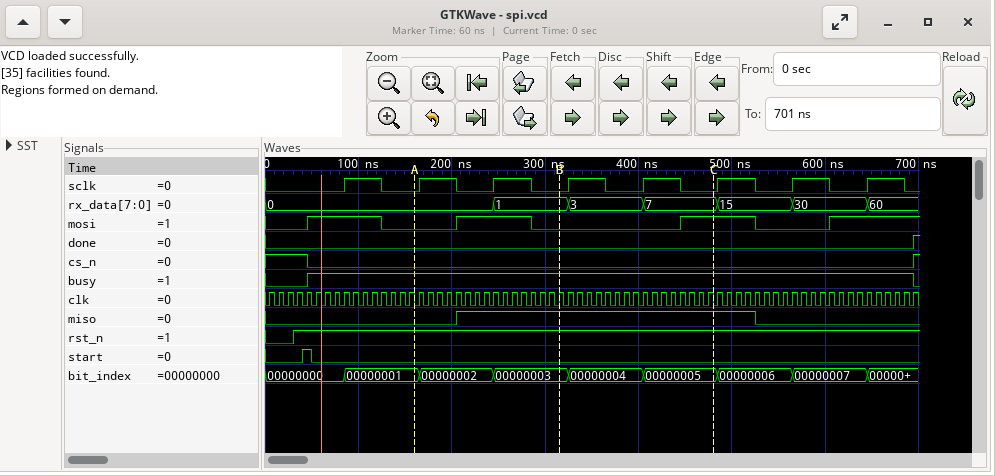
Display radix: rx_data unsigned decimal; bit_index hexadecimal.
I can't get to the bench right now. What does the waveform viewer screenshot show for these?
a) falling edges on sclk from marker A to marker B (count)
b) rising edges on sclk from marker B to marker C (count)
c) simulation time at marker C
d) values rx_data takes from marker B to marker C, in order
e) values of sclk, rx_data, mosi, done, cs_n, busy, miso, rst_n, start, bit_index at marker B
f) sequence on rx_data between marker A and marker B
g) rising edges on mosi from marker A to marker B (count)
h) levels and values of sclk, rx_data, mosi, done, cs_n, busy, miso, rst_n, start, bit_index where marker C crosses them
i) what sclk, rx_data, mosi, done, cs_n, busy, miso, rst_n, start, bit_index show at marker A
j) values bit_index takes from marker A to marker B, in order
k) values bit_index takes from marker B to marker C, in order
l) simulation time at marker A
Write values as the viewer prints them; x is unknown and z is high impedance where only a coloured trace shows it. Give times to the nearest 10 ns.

2
2
480 ns
1, 3, 7
sclk=0, rx_data=1, mosi=0, done=0, cs_n=0, busy=1, miso=1, rst_n=1, start=0, bit_index=00000003
0, 1
1
sclk=0, rx_data=7, mosi=1, done=0, cs_n=0, busy=1, miso=1, rst_n=1, start=0, bit_index=00000005
sclk=0, rx_data=0, mosi=0, done=0, cs_n=0, busy=1, miso=0, rst_n=1, start=0, bit_index=00000001
00000001, 00000002, 00000003
00000003, 00000004, 00000005
160 ns
